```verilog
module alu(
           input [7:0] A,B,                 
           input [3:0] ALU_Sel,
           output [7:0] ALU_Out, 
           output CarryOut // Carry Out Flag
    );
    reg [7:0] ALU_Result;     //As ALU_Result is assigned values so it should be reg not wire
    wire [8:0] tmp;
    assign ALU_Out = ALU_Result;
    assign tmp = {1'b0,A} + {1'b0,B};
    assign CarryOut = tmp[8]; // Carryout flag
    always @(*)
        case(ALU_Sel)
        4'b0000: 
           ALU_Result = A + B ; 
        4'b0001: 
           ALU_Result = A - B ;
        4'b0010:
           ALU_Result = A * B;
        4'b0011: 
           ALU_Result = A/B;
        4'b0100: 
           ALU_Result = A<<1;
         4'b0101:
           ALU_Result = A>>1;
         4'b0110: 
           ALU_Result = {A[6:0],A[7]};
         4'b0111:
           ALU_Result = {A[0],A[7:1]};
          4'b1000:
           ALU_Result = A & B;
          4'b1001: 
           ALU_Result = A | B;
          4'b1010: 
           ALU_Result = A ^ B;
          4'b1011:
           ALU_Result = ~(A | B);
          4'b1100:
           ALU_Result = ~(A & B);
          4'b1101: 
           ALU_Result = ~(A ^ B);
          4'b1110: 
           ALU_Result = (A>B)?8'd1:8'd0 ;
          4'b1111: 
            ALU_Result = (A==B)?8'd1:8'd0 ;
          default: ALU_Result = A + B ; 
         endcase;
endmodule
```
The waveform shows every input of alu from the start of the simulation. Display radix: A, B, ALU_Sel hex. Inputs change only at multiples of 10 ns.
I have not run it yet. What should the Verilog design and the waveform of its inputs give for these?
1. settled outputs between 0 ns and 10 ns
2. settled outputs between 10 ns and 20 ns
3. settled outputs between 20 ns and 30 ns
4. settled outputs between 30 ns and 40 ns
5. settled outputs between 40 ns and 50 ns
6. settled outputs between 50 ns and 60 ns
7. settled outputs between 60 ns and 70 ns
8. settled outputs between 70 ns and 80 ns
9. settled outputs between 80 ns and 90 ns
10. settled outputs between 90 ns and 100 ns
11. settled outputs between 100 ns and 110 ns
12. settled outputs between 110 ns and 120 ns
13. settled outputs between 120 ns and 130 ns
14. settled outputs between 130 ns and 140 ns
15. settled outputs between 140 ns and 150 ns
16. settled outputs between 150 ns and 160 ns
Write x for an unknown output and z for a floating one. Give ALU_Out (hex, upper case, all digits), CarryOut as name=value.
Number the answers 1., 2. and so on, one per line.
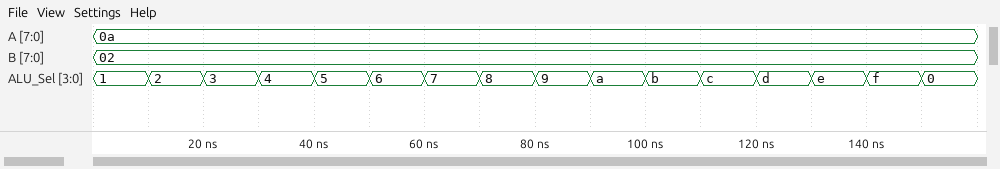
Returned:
1. ALU_Out=08, CarryOut=0
2. ALU_Out=14, CarryOut=0
3. ALU_Out=05, CarryOut=0
4. ALU_Out=14, CarryOut=0
5. ALU_Out=05, CarryOut=0
6. ALU_Out=14, CarryOut=0
7. ALU_Out=05, CarryOut=0
8. ALU_Out=02, CarryOut=0
9. ALU_Out=0A, CarryOut=0
10. ALU_Out=08, CarryOut=0
11. ALU_Out=F5, CarryOut=0
12. ALU_Out=FD, CarryOut=0
13. ALU_Out=F7, CarryOut=0
14. ALU_Out=01, CarryOut=0
15. ALU_Out=00, CarryOut=0
16. ALU_Out=0C, CarryOut=0
